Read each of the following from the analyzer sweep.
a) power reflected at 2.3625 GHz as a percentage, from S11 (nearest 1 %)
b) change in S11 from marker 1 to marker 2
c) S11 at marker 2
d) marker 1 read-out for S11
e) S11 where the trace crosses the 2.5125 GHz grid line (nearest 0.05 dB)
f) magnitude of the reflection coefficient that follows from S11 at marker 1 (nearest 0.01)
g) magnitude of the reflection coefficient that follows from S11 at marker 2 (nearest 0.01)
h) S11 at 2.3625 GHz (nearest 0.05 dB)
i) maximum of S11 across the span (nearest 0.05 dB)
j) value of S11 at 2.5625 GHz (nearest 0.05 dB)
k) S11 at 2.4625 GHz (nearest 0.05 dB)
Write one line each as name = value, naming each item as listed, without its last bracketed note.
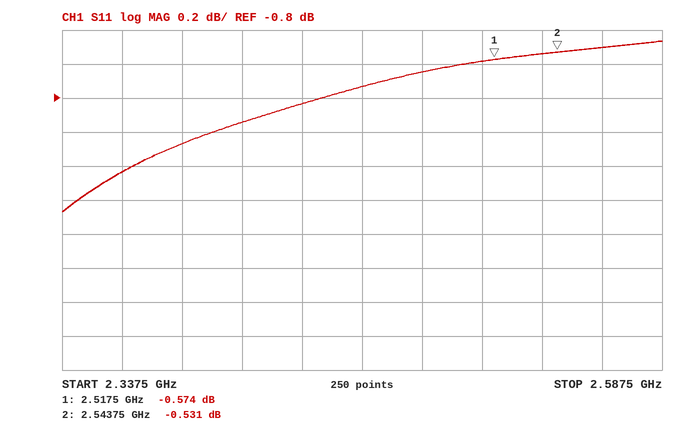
power reflected at 2.3625 GHz as a percentage, from S11 = 75 %
change in S11 from marker 1 to marker 2 = 0.043 dB
S11 at marker 2 = -0.531 dB
marker 1 read-out for S11 = -0.574 dB
S11 where the trace crosses the 2.5125 GHz grid line = -0.60 dB
magnitude of the reflection coefficient that follows from S11 at marker 1 = 0.94
magnitude of the reflection coefficient that follows from S11 at marker 2 = 0.94
S11 at 2.3625 GHz = -1.25 dB
maximum of S11 across the span = -0.45 dB
value of S11 at 2.5625 GHz = -0.50 dB
S11 at 2.4625 GHz = -0.75 dB
